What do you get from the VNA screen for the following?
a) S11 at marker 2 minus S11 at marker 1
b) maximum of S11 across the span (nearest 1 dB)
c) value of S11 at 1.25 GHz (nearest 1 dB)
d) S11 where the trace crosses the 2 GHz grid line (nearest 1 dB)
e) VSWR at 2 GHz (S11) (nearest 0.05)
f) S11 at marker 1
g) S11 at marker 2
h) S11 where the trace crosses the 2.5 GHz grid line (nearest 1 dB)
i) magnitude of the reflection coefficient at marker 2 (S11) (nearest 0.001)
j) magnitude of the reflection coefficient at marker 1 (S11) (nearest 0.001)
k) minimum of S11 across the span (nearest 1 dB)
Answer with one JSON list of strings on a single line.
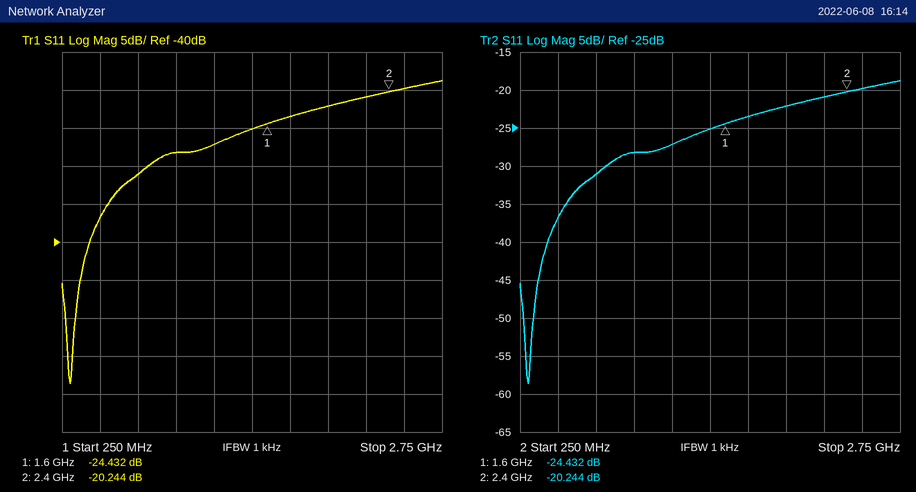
["4.188 dB", "-19 dB", "-27 dB", "-22 dB", "1.15", "-24.432 dB", "-20.244 dB", "-20 dB", "0.097", "0.060", "-59 dB"]
